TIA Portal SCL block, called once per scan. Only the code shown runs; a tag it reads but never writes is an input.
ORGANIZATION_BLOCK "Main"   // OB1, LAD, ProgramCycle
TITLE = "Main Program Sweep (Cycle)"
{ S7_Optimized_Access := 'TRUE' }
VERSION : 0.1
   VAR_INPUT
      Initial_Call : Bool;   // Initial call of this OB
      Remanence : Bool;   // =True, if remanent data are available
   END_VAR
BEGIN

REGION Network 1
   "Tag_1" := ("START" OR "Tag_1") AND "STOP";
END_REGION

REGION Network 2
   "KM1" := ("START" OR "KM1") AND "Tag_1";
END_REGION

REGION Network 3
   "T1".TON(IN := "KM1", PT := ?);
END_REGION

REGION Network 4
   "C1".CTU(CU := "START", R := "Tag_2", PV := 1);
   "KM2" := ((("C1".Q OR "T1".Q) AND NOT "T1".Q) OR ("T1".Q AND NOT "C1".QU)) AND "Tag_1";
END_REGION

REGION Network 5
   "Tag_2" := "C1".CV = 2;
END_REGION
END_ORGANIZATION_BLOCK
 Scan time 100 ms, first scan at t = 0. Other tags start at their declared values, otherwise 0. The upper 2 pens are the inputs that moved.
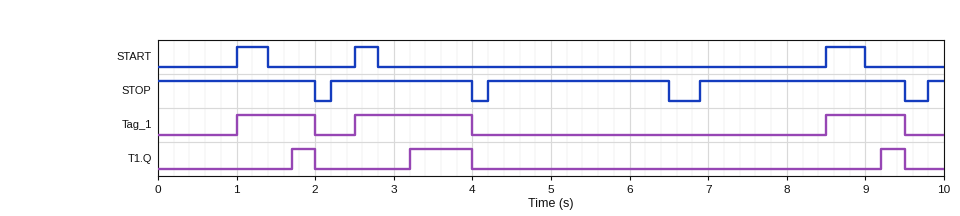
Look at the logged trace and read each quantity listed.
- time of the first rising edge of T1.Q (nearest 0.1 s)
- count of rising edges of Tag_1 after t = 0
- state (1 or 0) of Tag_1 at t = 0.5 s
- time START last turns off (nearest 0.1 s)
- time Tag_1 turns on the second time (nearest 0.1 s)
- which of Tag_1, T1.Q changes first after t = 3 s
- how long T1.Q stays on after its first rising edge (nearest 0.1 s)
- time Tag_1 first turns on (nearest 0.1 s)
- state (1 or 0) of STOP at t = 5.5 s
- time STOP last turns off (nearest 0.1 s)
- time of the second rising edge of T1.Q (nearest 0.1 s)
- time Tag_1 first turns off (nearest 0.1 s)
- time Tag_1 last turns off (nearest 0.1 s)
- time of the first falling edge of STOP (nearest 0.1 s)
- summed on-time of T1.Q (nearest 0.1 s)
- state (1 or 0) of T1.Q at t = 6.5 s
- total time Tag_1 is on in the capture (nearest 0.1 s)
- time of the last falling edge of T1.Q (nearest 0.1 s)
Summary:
1.7 s
3
0
9.0 s
2.5 s
T1.Q
0.3 s
1.0 s
1
9.5 s
3.2 s
2.0 s
9.5 s
2.0 s
1.4 s
0
3.5 s
9.5 s
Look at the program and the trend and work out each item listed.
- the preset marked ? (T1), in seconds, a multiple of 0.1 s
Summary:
0.7 s
